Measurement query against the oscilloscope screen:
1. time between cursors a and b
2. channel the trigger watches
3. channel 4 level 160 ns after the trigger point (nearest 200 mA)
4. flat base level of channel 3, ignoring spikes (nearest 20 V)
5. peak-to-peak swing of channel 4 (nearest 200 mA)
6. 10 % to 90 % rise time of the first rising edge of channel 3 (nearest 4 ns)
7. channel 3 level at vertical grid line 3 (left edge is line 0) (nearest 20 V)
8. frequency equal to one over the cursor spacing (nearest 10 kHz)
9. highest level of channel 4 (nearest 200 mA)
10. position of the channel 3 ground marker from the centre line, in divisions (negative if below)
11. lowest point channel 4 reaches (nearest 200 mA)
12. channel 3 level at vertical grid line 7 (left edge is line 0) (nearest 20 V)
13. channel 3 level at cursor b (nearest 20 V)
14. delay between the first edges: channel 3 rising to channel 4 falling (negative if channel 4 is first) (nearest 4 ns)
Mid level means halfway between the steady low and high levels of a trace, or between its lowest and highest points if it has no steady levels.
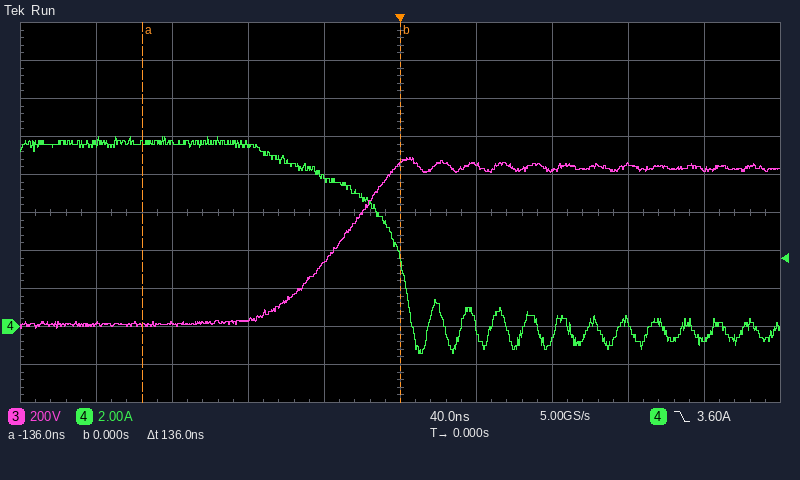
136 ns
channel 4
-600 mA
20 V
11.4 A
56 ns
40 V
7.35 MHz
10.0 A
-3.0 div
-1.4 A
820 V
860 V
+32 ns
